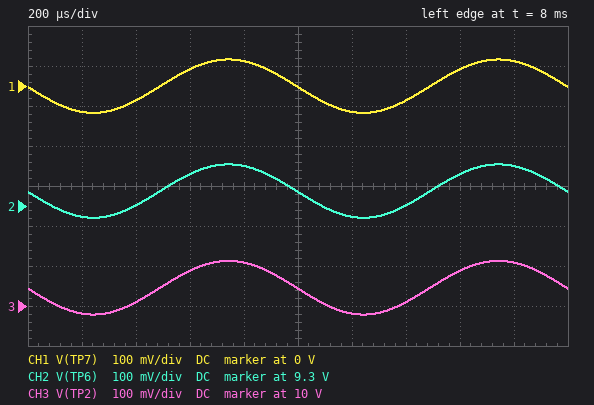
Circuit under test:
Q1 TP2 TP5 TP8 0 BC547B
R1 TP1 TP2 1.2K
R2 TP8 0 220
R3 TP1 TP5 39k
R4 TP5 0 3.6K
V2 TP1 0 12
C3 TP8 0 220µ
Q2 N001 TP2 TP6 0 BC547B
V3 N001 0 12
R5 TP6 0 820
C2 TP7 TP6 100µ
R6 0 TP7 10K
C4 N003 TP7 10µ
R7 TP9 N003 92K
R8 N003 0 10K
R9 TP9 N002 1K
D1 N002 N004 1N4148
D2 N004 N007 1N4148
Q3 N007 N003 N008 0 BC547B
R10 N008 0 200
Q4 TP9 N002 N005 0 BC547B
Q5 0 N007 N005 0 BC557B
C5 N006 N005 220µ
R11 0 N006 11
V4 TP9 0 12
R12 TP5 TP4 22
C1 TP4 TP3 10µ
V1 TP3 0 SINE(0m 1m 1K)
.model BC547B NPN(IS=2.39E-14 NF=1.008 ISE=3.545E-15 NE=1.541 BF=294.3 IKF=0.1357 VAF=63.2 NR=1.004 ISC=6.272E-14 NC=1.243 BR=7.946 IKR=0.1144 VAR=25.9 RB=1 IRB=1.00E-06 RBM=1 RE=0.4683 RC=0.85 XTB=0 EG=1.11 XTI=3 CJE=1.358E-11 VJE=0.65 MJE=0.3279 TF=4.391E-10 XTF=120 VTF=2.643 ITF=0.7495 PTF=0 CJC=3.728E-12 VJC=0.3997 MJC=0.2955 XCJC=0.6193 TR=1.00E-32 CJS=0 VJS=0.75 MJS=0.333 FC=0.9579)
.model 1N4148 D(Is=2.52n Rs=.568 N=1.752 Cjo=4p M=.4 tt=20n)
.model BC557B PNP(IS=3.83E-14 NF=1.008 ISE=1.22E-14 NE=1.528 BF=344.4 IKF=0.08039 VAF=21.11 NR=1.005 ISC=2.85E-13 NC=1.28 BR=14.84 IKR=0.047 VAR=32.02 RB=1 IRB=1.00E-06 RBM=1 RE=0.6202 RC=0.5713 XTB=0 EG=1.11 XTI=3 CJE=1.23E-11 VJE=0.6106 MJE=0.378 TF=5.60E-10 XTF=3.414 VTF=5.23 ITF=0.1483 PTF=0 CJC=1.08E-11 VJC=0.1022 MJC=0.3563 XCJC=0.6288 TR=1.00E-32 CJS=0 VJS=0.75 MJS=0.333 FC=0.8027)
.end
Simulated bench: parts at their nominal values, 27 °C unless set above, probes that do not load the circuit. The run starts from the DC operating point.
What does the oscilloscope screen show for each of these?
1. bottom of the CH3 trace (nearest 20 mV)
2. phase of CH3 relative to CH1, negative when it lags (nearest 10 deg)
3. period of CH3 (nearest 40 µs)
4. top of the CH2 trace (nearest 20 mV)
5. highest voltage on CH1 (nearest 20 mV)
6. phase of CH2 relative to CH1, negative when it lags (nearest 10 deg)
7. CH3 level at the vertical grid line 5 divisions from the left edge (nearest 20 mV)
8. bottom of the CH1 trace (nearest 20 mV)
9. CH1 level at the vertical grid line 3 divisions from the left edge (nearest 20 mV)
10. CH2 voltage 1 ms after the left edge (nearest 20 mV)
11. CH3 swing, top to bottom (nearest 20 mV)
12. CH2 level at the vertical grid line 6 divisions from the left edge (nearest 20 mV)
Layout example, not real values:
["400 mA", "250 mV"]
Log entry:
["9.98 V", "0 deg", "1.00 ms", "9.40 V", "60 mV", "0 deg", "10.04 V", "-60 mV", "40 mV", "9.34 V", "140 mV", "9.28 V"]
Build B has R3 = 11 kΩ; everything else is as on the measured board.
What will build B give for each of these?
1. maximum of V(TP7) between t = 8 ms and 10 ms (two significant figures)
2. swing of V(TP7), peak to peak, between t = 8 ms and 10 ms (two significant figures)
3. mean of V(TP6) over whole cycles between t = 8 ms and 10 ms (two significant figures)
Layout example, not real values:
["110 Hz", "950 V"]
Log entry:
["4.8 mV", "8.7 mV", "1.3 V"]
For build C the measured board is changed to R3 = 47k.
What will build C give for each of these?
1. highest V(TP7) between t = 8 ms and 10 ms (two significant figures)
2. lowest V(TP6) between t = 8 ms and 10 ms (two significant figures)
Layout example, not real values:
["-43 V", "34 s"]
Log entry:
["41 mV", "10 V"]
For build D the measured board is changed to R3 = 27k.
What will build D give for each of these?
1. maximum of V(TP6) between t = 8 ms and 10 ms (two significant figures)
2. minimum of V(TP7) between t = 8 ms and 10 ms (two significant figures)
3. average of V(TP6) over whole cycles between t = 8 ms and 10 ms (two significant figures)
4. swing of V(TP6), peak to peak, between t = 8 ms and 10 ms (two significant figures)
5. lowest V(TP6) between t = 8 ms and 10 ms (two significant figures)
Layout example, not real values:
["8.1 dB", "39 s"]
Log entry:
["7.5 V", "-130 mV", "7.4 V", "250 mV", "7.3 V"]
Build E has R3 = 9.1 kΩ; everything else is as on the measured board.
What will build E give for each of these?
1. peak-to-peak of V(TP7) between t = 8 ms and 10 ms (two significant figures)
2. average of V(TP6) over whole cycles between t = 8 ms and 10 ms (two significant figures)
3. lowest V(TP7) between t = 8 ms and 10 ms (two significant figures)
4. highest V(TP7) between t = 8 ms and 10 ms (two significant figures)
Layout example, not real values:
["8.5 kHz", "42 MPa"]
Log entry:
["3.2 mV", "1.3 V", "-1.5 mV", "1.7 mV"]
